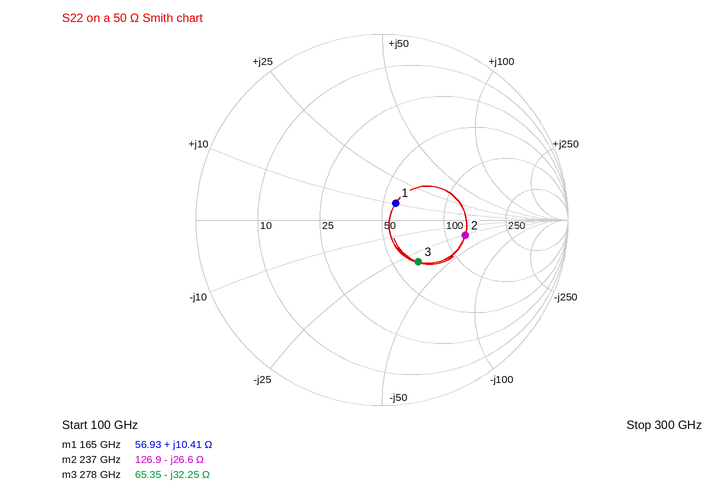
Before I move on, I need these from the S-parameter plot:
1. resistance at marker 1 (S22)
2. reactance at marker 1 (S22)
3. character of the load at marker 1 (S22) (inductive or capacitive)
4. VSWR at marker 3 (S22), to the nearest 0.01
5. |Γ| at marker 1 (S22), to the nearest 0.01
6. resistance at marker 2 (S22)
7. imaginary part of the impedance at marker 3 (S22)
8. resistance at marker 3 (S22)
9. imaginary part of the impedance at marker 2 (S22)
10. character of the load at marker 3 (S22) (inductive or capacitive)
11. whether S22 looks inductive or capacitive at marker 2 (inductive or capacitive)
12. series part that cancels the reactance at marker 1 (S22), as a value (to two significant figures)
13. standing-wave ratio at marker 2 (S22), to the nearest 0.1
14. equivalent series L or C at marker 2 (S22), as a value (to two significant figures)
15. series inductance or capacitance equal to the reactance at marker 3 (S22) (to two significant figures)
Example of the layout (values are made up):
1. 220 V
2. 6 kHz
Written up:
1. 56.93 Ω
2. +10.41 Ω
3. inductive
4. 1.85
5. 0.12
6. 126.9 Ω
7. -32.25 Ω
8. 65.35 Ω
9. -26.6 Ω
10. capacitive
11. capacitive
12. 93 fF
13. 2.7
14. 25 fF
15. 18 fF
